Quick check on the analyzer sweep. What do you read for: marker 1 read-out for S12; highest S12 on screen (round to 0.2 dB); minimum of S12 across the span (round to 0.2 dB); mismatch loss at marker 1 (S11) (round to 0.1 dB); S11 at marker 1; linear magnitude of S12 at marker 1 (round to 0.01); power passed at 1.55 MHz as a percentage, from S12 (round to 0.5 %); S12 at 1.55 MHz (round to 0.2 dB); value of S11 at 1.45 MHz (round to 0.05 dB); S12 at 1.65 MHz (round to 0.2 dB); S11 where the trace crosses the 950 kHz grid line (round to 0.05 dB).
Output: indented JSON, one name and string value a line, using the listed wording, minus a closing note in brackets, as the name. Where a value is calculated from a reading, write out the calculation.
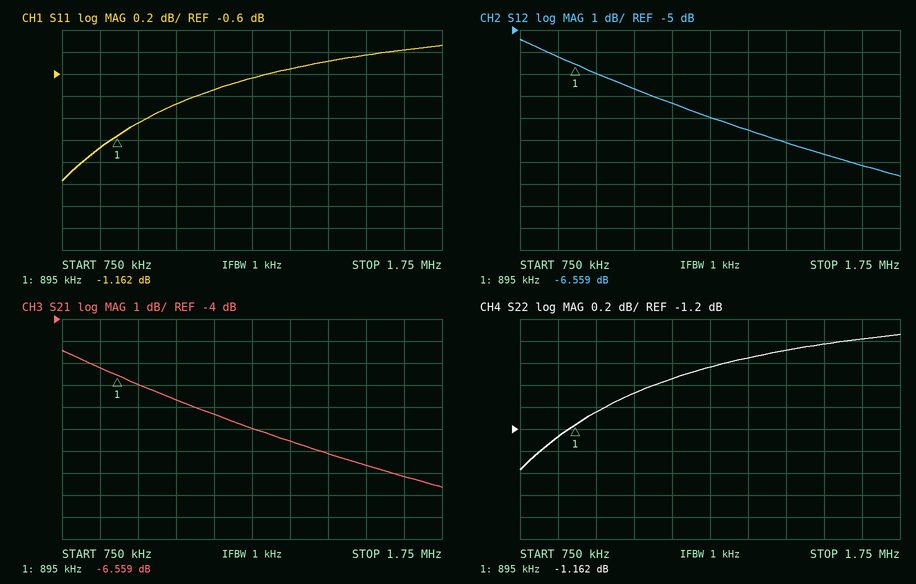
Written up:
{
  "marker 1 read-out for S12": "-6.559 dB",
  "highest S12 on screen": "-5.4 dB",
  "minimum of S12 across the span": "-11.6 dB",
  "mismatch loss at marker 1 (S11)": "−10 log10(1 − 10^(-1.162/10)) ≈ 6.3 dB",
  "S11 at marker 1": "-1.162 dB",
  "linear magnitude of S12 at marker 1": "10^(-6.559/20) ≈ 0.47",
  "power passed at 1.55 MHz as a percentage, from S12": "10^(-10.6/10) ≈ 8.71 %, so 8.5 % to the nearest 0.5 %",
  "S12 at 1.55 MHz": "-10.6 dB",
  "value of S11 at 1.45 MHz": "-0.50 dB",
  "S12 at 1.65 MHz": "-11.2 dB",
  "S11 where the trace crosses the 950 kHz grid line": "-1.05 dB"
}
